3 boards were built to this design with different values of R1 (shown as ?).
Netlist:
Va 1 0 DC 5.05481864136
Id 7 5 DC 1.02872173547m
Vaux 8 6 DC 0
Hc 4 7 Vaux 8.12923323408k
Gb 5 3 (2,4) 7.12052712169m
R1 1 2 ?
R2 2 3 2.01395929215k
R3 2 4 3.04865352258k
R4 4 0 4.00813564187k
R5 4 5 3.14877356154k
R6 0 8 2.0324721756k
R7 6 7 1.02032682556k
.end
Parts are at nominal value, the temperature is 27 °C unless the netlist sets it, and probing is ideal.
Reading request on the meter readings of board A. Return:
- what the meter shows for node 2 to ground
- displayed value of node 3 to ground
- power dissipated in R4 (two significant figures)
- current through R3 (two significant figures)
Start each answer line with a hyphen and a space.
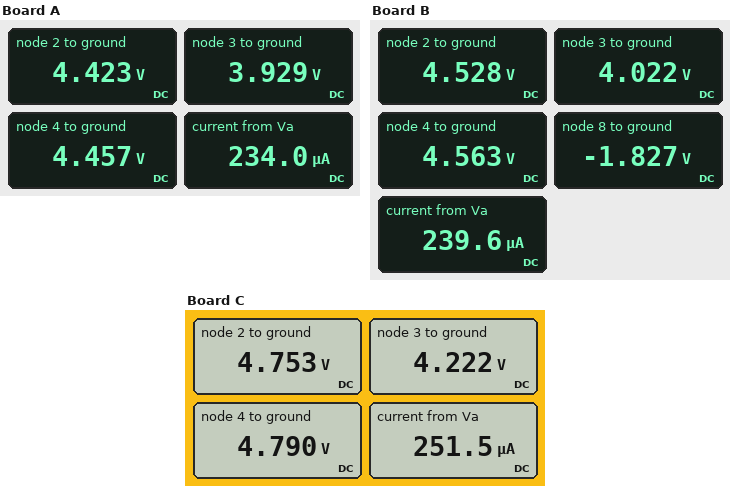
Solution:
- 4.423 V
- 3.929 V
- 5.0 mW
- 11 µA
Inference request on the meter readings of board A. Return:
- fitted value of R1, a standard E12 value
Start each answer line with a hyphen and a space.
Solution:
- 2.7 kΩ
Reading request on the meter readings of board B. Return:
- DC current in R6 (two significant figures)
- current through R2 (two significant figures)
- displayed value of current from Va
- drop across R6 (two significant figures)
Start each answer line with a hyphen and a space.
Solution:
- 900 µA
- 250 µA
- 239.6 µA
- 1.8 V
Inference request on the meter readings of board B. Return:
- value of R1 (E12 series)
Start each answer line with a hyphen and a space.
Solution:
- 2.2 kΩ
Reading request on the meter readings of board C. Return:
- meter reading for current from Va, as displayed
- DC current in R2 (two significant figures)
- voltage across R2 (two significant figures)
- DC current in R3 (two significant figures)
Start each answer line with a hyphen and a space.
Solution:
- 251.5 µA
- 260 µA
- 530 mV
- 12 µA
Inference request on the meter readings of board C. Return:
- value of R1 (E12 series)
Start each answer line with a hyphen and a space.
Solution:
- 1.2 kΩ
